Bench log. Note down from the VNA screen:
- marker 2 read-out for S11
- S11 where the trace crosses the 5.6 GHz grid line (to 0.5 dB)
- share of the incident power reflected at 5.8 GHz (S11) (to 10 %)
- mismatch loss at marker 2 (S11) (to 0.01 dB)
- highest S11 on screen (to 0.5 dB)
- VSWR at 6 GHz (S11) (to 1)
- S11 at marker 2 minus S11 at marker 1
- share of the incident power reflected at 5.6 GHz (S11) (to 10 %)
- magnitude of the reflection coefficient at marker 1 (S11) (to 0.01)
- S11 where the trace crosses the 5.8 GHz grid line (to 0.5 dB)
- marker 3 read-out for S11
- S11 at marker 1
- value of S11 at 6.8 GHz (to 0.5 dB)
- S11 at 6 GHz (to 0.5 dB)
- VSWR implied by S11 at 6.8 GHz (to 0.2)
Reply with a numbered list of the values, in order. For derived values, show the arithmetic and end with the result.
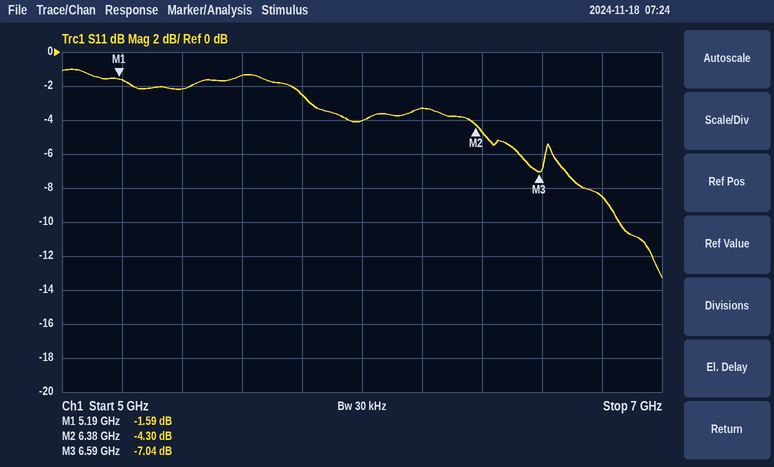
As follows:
1. -4.30 dB
2. -1.5 dB
3. 10^(-2.5/10) ≈ 56.2 %, so 60 % to the nearest 10 %
4. −10 log10(1 − 10^(-4.3/10)) ≈ 2.02 dB
5. -1.0 dB
6. |Γ| = 10^(-4/20) = 0.6310; VSWR = (1 + 0.6310)/(1 − 0.6310) ≈ 4
7. -4.3 − (-1.59) = -2.71 dB
8. 10^(-1.5/10) ≈ 70.8 %, so 70 % to the nearest 10 %
9. 10^(-1.59/20) ≈ 0.83
10. -2.5 dB
11. -7.04 dB
12. -1.59 dB
13. -8.5 dB
14. -4.0 dB
15. |Γ| = 10^(-8.5/20) = 0.3758; VSWR = (1 + 0.3758)/(1 − 0.3758) ≈ 2.2
